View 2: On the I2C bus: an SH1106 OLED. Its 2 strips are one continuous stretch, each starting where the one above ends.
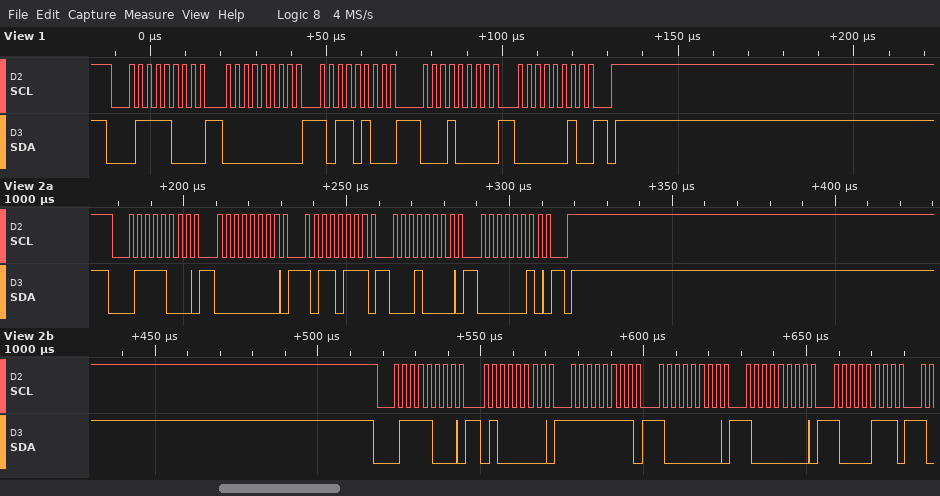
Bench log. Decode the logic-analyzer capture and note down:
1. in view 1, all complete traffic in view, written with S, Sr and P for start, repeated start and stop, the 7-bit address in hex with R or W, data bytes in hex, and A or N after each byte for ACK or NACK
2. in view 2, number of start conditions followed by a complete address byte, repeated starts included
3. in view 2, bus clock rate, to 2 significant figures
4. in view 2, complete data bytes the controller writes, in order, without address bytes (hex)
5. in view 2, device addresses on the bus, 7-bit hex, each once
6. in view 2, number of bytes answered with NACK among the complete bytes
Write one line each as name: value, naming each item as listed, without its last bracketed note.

in view 1, all complete traffic in view, written with S, Sr and P for start, repeated start and stop, the 7-bit address in hex with R or W, data bytes in hex, and A or N after each byte for ACK or NACK: S 3CW A 00 A B4 A 10 A 02 A P
in view 2, number of start conditions followed by a complete address byte, repeated starts included: 2
in view 2, bus clock rate, to 2 significant figures: 400 kHz
in view 2, complete data bytes the controller writes, in order, without address bytes: 00 B7 10 02 40 FF 80 80 87
in view 2, device addresses on the bus, 7-bit hex, each once: 0x3C
in view 2, number of bytes answered with NACK among the complete bytes: 0
